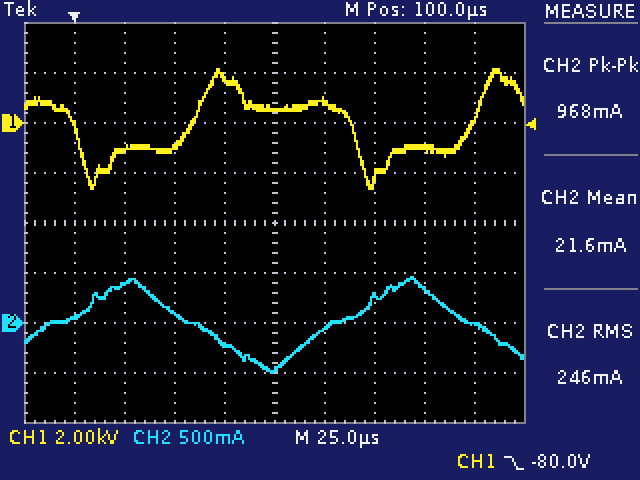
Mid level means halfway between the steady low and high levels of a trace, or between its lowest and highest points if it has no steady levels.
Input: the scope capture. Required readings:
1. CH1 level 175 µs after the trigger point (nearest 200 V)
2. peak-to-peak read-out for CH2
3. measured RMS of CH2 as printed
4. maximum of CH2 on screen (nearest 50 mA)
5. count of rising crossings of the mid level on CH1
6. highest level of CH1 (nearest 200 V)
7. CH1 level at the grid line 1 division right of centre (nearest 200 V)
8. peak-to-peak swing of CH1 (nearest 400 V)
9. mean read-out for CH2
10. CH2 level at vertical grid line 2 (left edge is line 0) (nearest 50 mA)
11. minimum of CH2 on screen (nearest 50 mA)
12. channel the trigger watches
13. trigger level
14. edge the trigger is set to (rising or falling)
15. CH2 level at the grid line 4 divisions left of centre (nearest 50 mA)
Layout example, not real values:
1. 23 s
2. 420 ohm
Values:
1. -1.0 kV
2. 968 mA
3. 246 mA
4. 450 mA
5. 2
6. 2.2 kV
7. 800 V
8. 4.8 kV
9. 21.6 mA
10. 400 mA
11. -500 mA
12. CH1
13. -80.0 V
14. falling
15. 50 mA
